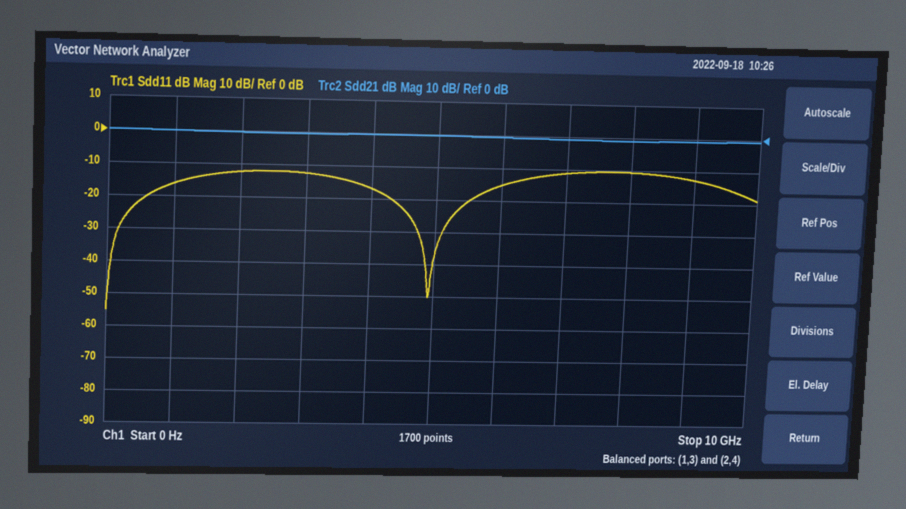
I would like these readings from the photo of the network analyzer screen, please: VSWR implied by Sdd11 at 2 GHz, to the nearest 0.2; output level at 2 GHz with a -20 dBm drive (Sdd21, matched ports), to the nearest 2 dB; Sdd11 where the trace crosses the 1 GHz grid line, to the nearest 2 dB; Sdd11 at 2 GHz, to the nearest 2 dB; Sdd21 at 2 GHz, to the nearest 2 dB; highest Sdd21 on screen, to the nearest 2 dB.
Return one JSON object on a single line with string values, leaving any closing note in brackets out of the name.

{"VSWR implied by Sdd11 at 2 GHz, to the nearest 0.2": "1.6", "output level at 2 GHz with a -20 dBm drive (Sdd21, matched ports), to the nearest 2 dB": "-20 dBm", "Sdd11 where the trace crosses the 1 GHz grid line, to the nearest 2 dB": "-16 dB", "Sdd11 at 2 GHz, to the nearest 2 dB": "-12 dB", "Sdd21 at 2 GHz, to the nearest 2 dB": "0 dB", "highest Sdd21 on screen, to the nearest 2 dB": "0 dB"}
